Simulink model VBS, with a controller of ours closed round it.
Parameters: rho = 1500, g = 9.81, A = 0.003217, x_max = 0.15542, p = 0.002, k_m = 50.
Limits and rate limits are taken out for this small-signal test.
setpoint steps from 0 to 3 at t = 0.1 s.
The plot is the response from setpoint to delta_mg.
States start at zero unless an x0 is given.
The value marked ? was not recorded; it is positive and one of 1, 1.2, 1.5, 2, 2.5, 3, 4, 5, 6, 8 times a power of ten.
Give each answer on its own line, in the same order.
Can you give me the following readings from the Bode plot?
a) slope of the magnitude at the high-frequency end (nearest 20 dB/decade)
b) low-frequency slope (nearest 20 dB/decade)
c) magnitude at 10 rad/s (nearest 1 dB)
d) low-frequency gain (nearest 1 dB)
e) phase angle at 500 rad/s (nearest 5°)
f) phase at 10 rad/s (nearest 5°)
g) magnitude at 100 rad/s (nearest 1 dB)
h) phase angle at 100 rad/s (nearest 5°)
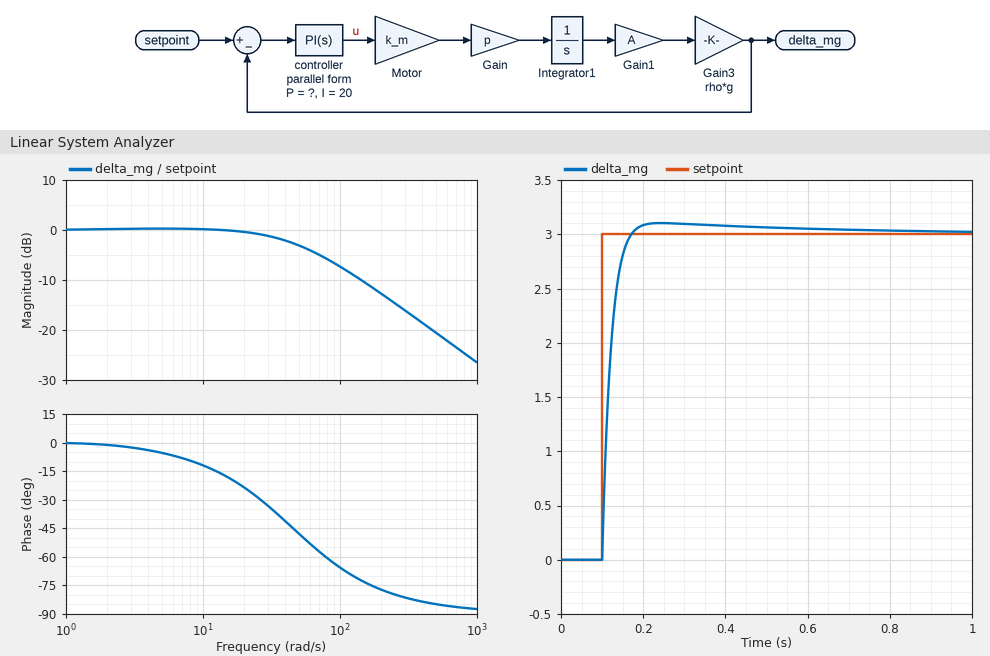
-20 dB/decade
0 dB/decade
0 dB
0 dB
-85°
-10°
-7 dB
-65°
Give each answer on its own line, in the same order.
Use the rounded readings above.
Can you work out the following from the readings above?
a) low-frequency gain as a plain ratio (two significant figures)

1.0
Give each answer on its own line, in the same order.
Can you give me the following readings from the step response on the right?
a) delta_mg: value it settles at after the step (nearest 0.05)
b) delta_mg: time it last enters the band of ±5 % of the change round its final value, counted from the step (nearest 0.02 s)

3.00
0.06 s
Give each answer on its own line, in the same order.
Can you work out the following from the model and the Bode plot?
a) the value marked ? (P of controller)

10
